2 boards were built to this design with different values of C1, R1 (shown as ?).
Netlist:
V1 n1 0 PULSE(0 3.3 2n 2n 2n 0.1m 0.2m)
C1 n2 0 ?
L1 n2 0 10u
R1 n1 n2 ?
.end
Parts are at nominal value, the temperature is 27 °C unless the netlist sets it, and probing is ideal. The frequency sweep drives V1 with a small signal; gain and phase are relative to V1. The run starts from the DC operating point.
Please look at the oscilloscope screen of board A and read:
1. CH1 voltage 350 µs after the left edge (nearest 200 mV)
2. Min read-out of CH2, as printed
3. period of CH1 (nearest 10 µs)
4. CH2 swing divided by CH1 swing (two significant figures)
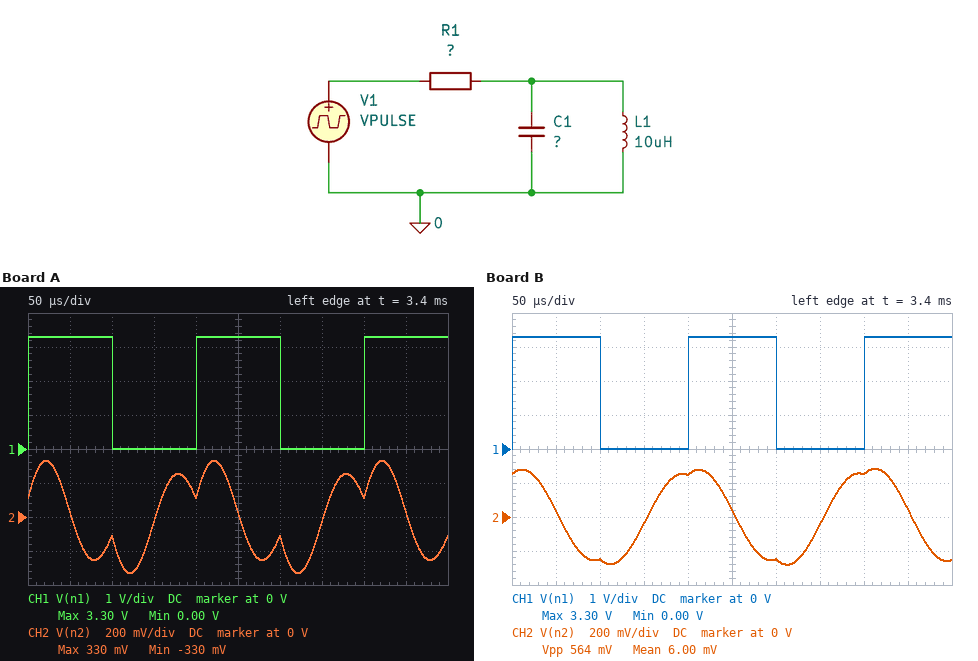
0 V
-330 mV
200 µs
0.20
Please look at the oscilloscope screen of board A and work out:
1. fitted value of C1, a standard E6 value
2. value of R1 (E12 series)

33 µF
3.3 Ω
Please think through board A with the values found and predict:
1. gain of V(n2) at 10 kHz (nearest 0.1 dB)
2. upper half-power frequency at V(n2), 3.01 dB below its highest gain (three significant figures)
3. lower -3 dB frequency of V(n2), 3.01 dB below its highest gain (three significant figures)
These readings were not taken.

-5.5 dB
9.52 kHz
8.06 kHz
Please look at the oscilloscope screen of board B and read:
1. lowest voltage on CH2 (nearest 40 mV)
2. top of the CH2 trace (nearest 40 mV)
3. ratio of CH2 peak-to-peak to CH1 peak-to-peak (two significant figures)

-280 mV
280 mV
0.17
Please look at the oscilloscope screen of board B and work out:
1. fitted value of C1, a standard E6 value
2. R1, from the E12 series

68 µF
6.8 Ω
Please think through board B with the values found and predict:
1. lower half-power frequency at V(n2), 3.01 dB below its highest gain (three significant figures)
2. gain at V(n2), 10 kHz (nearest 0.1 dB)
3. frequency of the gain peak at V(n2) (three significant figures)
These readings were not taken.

5.93 kHz
-25.2 dB
6.10 kHz
